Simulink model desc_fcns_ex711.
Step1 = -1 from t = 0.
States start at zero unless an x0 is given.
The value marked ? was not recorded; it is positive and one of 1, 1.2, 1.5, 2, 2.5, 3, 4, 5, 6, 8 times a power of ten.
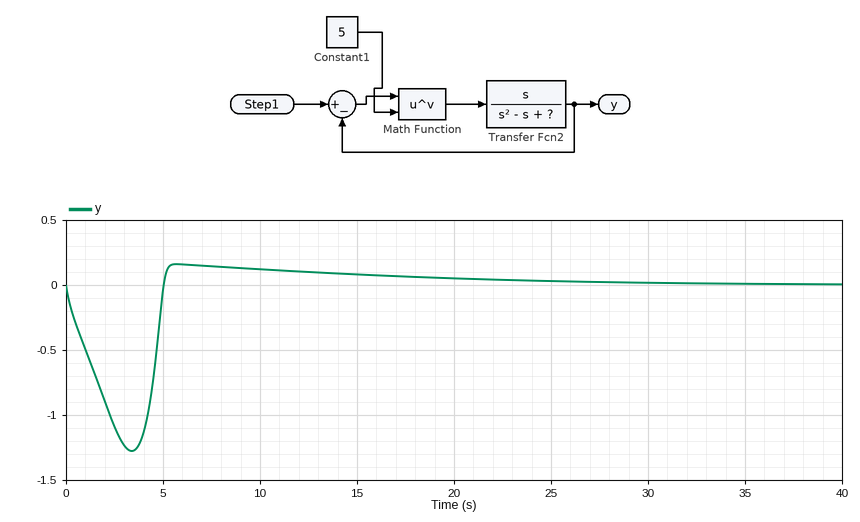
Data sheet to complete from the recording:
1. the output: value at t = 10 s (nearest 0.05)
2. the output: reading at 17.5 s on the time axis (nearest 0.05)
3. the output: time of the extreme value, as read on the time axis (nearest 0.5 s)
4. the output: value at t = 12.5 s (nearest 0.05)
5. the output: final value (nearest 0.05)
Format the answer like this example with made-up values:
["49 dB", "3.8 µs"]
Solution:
["0.10", "0.05", "3.5 s", "0.10", "0.00"]
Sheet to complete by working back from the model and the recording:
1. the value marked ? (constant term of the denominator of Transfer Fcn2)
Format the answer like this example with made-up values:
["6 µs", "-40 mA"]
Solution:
["0.5"]
